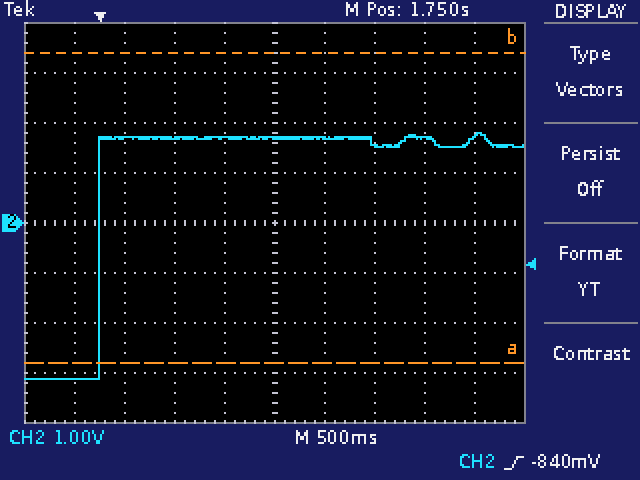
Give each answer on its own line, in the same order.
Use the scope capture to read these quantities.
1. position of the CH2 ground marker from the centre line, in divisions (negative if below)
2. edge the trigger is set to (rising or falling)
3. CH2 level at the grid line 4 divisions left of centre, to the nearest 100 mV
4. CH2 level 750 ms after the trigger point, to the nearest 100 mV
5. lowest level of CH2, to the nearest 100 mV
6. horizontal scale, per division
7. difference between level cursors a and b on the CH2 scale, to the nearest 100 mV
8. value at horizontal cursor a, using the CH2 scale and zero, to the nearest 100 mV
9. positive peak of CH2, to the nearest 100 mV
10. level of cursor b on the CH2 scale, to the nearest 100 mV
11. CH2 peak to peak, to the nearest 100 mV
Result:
0.0 div
rising
-3.1 V
1.7 V
-3.1 V
500 ms
6.2 V
-2.8 V
1.8 V
3.4 V
4.9 V
